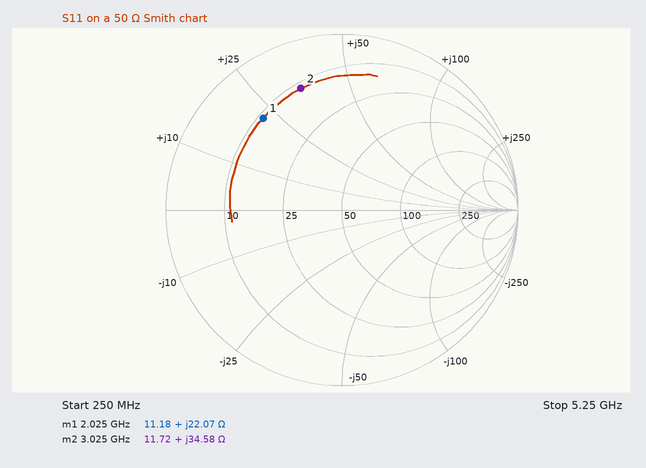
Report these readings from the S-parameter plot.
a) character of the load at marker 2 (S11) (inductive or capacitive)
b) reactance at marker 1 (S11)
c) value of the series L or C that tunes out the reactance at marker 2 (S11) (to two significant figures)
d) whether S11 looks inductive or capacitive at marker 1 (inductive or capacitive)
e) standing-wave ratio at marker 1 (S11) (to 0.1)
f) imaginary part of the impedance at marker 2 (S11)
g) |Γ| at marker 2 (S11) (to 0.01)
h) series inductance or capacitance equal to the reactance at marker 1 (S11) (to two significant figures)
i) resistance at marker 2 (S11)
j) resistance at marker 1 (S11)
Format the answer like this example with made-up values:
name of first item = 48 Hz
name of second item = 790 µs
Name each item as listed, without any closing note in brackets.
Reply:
character of the load at marker 2 (S11) = inductive
reactance at marker 1 = +22.07 Ω
value of the series L or C that tunes out the reactance at marker 2 (S11) = 1.5 pF
whether S11 looks inductive or capacitive at marker 1 = inductive
standing-wave ratio at marker 1 (S11) = 5.4
imaginary part of the impedance at marker 2 = +34.58 Ω
|Γ| at marker 2 (S11) = 0.73
series inductance or capacitance equal to the reactance at marker 1 (S11) = 1.7 nH
resistance at marker 2 = 11.72 Ω
resistance at marker 1 = 11.18 Ω
